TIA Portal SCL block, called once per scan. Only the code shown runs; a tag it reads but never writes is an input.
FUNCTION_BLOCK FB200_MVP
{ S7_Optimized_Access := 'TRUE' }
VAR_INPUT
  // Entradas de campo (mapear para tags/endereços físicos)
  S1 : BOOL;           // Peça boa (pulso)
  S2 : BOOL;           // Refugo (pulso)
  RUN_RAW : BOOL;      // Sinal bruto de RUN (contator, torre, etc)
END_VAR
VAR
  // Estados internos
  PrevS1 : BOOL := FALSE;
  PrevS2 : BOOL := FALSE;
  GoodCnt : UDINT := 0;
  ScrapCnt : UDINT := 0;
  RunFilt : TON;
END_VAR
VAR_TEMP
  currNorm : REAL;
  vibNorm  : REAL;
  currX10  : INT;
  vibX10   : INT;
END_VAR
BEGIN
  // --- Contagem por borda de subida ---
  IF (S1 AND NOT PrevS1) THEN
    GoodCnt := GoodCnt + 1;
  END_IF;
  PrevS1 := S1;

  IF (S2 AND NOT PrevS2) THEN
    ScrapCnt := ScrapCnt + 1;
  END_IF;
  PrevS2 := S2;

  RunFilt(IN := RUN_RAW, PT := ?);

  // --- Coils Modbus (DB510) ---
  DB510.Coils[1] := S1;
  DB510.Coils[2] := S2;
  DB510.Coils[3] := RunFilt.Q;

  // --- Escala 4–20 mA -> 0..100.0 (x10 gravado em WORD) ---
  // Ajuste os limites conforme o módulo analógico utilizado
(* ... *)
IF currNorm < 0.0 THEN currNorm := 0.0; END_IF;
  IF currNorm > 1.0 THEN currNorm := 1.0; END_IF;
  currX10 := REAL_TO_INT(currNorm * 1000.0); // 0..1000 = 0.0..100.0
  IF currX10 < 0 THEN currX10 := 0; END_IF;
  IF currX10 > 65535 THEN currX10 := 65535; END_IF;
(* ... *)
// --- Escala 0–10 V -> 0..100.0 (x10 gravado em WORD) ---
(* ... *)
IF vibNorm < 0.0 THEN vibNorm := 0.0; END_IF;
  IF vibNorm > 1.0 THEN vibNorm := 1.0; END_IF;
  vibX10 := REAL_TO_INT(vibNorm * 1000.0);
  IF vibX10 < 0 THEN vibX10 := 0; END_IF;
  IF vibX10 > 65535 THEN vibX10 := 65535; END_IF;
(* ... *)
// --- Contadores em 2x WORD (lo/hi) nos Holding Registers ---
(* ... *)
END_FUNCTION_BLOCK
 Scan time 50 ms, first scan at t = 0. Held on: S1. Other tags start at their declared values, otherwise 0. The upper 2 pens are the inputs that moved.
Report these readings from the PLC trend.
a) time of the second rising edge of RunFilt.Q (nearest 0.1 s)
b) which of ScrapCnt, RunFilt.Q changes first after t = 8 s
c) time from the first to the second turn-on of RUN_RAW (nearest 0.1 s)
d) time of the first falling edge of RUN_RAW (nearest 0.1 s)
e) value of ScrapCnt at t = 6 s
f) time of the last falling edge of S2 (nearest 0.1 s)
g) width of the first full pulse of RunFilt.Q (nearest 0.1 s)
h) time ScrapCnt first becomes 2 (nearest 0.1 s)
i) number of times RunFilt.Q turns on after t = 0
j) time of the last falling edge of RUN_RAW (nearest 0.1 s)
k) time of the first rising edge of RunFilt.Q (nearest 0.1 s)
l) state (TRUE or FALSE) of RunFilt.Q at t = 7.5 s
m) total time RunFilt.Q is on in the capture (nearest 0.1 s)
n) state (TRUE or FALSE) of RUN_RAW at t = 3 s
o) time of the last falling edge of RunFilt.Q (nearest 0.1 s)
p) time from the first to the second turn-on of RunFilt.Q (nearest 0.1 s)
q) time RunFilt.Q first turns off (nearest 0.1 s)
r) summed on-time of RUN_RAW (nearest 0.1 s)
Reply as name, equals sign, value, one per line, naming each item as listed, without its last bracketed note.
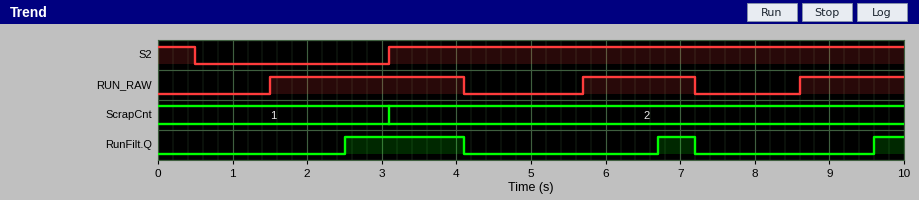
time of the second rising edge of RunFilt.Q = 6.7 s
which of ScrapCnt, RunFilt.Q changes first after t = 8 s = RunFilt.Q
time from the first to the second turn-on of RUN_RAW = 4.2 s
time of the first falling edge of RUN_RAW = 4.1 s
value of ScrapCnt at t = 6 s = 2
time of the last falling edge of S2 = 0.5 s
width of the first full pulse of RunFilt.Q = 1.6 s
time ScrapCnt first becomes 2 = 3.1 s
number of times RunFilt.Q turns on after t = 0 = 3
time of the last falling edge of RUN_RAW = 7.2 s
time of the first rising edge of RunFilt.Q = 2.5 s
state (TRUE or FALSE) of RunFilt.Q at t = 7.5 s = FALSE
total time RunFilt.Q is on in the capture = 2.5 s
state (TRUE or FALSE) of RUN_RAW at t = 3 s = TRUE
time of the last falling edge of RunFilt.Q = 7.2 s
time from the first to the second turn-on of RunFilt.Q = 4.2 s
time RunFilt.Q first turns off = 4.1 s
summed on-time of RUN_RAW = 5.5 s
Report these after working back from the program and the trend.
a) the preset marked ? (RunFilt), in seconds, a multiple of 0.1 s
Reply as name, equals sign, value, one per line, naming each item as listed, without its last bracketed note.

the preset marked ? (RunFilt), in seconds, a multiple of 0.1 s = 1.0 s
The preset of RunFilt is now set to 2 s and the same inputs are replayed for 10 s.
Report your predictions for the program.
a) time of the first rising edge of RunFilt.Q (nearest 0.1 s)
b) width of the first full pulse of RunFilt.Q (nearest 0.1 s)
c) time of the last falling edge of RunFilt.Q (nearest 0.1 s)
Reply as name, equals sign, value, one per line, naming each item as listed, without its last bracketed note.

time of the first rising edge of RunFilt.Q = 3.5 s
width of the first full pulse of RunFilt.Q = 0.6 s
time of the last falling edge of RunFilt.Q = 4.1 s
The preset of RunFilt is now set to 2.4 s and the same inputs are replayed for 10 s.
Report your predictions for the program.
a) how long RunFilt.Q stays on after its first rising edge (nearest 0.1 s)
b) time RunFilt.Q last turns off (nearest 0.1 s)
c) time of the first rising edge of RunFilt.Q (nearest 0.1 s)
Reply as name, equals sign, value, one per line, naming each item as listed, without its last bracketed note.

how long RunFilt.Q stays on after its first rising edge = 0.2 s
time RunFilt.Q last turns off = 4.1 s
time of the first rising edge of RunFilt.Q = 3.9 s
